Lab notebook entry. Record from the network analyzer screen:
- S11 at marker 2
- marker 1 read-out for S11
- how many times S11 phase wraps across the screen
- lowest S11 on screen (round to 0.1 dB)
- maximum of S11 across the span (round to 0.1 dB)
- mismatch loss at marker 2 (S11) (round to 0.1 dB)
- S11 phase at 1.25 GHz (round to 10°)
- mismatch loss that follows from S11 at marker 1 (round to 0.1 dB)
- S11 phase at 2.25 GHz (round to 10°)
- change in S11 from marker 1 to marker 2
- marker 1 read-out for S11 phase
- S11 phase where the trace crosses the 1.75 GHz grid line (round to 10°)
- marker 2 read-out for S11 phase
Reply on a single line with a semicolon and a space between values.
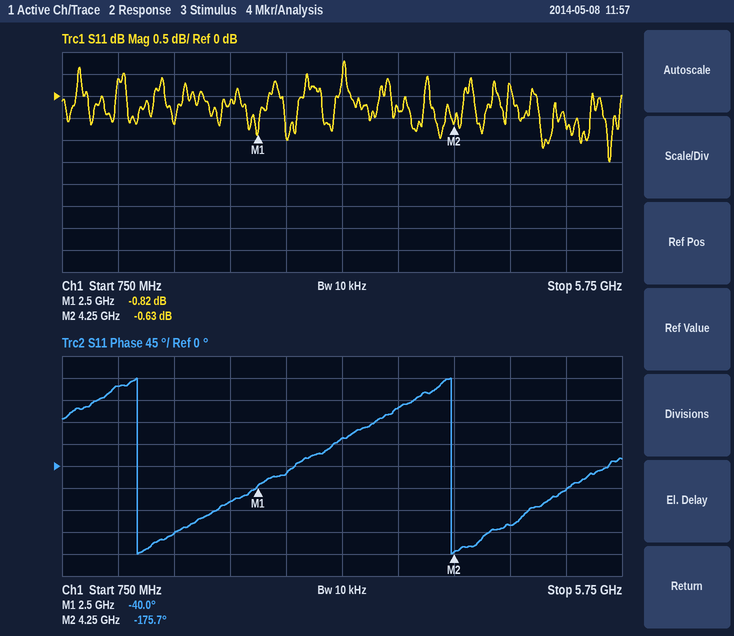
-0.63 dB; -0.82 dB; 2; -1.5 dB; 0.8 dB; 8.7 dB; 160°; 7.6 dB; -70°; 0.19 dB; -40.0°; -140°; -175.7°
